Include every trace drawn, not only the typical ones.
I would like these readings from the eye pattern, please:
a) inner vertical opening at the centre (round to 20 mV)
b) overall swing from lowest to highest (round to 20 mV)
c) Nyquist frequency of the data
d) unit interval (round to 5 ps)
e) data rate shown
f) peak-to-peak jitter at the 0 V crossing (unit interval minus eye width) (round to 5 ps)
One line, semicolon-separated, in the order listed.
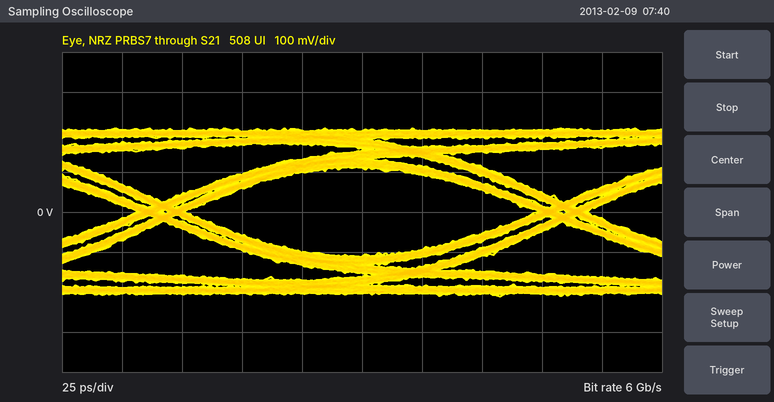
220 mV; 420 mV; 3 GHz; 165 ps; 6 Gb/s; 20 ps
